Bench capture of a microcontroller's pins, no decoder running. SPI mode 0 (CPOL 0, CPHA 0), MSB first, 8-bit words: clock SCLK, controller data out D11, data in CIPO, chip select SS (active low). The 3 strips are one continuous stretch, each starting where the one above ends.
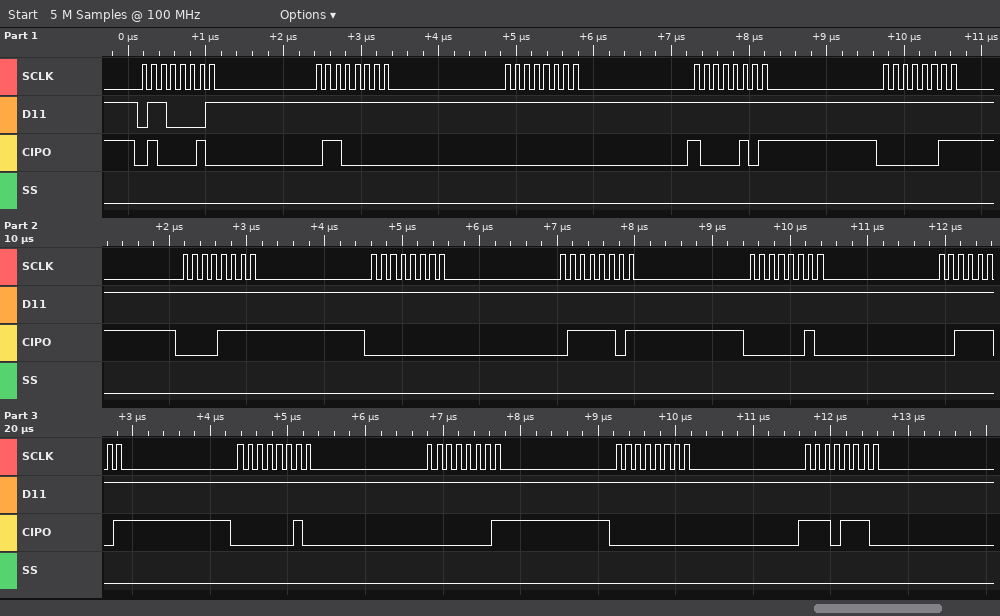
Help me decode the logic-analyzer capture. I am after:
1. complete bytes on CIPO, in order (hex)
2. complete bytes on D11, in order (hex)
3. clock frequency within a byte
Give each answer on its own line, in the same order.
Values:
0x42 0x60 0x00 0x85 0x03 0x0F 0x00 0x7D 0x02 0x3D 0x02 0x01 0x00 0xEE
0x61 0xFF 0xFF 0xFF 0xFF 0xFF 0xFF 0xFF 0xFF 0xFF 0xFF 0xFF 0xFF 0xFF
8 MHz
